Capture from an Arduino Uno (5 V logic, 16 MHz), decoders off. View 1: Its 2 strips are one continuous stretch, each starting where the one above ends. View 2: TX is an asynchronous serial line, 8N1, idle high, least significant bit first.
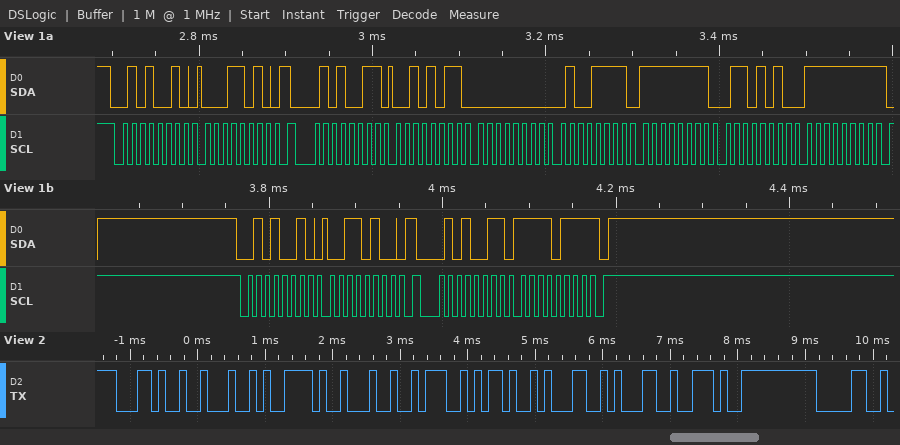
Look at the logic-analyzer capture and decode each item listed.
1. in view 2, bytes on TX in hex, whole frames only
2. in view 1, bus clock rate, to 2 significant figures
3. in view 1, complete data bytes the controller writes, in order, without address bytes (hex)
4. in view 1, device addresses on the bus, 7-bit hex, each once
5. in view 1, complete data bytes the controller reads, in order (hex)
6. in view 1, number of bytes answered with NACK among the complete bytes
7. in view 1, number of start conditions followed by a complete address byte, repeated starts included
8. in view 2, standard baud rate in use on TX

2C 22 79 22 3A 2D 31 31 2E 30
100 kHz
1A 34
0x29
2B 00 4F FF 6A FF F7
2
4
9600 baud
